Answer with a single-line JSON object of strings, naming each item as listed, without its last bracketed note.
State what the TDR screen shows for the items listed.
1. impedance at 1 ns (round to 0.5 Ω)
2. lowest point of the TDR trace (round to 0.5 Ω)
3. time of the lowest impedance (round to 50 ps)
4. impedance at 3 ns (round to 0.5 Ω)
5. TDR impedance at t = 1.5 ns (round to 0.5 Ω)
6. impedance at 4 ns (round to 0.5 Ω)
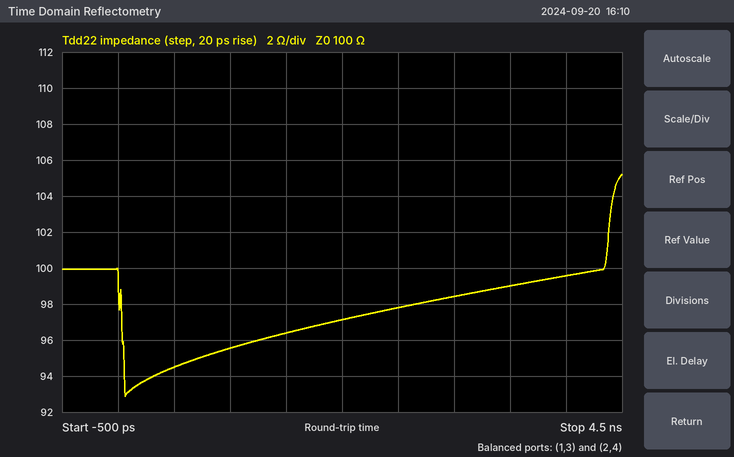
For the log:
{"impedance at 1 ns": "95.5 Ω", "lowest point of the TDR trace": "93.0 Ω", "time of the lowest impedance": "50 ps", "impedance at 3 ns": "98.5 Ω", "TDR impedance at t = 1.5 ns": "96.5 Ω", "impedance at 4 ns": "99.5 Ω"}
